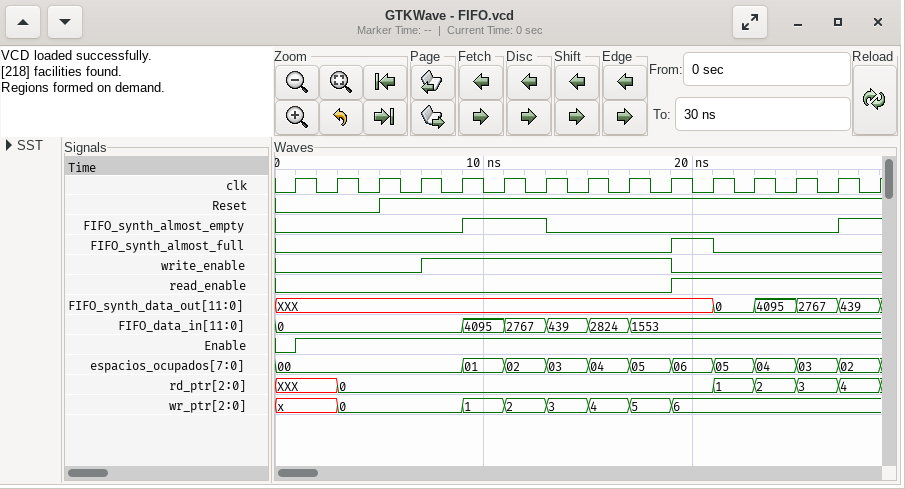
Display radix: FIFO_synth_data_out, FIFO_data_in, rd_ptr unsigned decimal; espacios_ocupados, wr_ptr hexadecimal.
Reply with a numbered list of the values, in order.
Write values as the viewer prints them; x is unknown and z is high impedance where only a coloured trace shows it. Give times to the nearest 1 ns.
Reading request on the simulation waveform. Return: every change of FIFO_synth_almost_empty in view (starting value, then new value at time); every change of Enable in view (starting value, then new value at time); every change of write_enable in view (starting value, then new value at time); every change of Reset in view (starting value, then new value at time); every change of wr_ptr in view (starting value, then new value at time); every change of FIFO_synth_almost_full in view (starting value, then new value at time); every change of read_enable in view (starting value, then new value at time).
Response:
1. 0, 1 at 9 ns, 0 at 13 ns, 1 at 27 ns
2. 0, 1 at 1 ns
3. 0, 1 at 7 ns, 0 at 19 ns
4. 0, 1 at 5 ns
5. x, 0 at 3 ns, 1 at 9 ns, 2 at 11 ns, 3 at 13 ns, 4 at 15 ns, 5 at 17 ns, 6 at 19 ns
6. 0, 1 at 19 ns, 0 at 21 ns
7. 0, 1 at 19 ns
